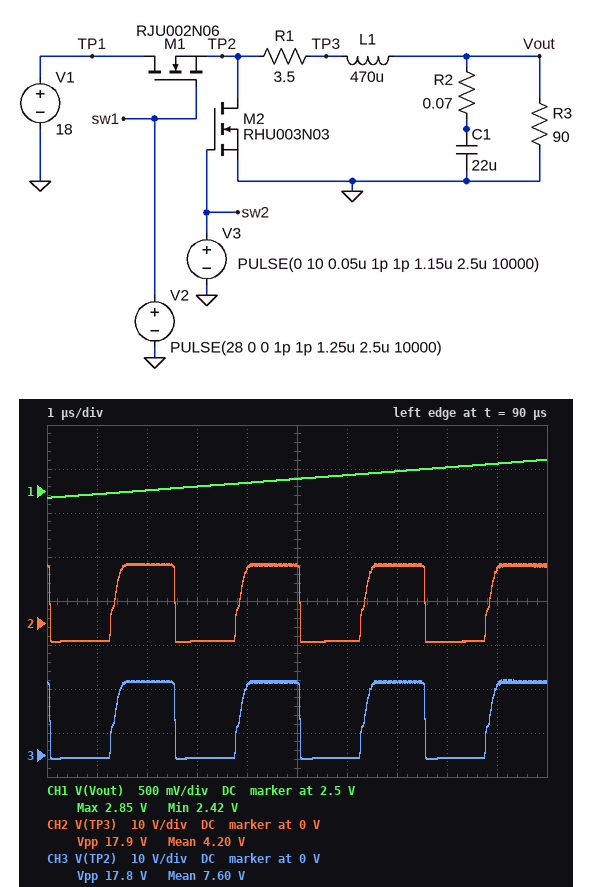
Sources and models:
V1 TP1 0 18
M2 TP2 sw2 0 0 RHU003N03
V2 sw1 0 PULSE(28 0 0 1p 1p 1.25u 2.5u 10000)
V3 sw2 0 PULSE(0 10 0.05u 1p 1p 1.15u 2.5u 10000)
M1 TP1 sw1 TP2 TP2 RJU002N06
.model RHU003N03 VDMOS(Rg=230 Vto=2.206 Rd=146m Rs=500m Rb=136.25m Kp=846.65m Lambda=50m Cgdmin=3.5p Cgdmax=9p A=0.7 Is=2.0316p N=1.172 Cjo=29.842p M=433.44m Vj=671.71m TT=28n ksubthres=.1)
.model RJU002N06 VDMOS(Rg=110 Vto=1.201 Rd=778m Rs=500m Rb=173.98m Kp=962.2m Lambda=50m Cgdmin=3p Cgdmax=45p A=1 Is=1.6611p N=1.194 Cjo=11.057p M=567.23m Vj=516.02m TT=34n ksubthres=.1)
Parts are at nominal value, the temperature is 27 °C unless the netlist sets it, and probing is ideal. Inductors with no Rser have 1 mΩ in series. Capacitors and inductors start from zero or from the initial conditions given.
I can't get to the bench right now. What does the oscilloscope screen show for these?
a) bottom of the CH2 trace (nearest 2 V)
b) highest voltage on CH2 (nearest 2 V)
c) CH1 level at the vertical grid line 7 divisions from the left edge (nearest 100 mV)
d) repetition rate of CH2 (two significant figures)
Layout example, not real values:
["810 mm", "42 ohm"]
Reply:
["-4 V", "14 V", "2.7 V", "400 kHz"]
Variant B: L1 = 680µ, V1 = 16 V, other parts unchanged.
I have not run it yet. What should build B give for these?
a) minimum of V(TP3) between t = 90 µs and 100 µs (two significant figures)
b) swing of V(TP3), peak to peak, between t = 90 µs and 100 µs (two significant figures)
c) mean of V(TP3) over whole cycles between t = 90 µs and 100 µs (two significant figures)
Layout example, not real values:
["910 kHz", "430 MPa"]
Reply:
["-3.4 V", "16 V", "4.5 V"]
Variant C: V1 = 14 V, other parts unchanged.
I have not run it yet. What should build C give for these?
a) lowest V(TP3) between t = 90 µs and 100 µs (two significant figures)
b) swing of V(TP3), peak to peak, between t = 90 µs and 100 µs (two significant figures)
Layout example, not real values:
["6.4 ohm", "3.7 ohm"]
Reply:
["-3.6 V", "14 V"]
